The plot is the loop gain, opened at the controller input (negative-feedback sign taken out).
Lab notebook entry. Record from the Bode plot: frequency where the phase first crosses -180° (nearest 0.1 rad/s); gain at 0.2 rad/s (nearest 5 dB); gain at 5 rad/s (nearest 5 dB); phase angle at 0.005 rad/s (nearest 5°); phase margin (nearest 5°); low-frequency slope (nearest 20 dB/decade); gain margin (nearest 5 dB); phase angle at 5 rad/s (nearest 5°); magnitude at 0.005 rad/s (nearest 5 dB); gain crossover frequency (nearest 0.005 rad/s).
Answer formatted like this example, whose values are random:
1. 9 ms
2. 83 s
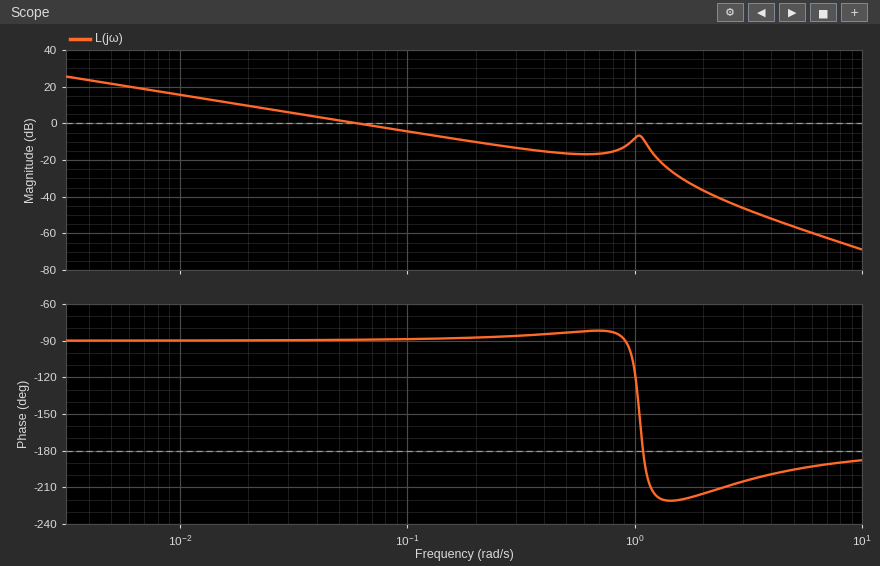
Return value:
1. 1.1 rad/s
2. -10 dB
3. -55 dB
4. -90°
5. 90°
6. -20 dB/decade
7. 10 dB
8. -195°
9. 20 dB
10. 0.060 rad/s
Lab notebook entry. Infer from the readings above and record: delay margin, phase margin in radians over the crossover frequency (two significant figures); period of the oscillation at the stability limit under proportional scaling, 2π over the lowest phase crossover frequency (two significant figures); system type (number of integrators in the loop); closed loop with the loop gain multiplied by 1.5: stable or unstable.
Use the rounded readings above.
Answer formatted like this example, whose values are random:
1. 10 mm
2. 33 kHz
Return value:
1. 26 s
2. 5.7 s
3. 1
4. stable
